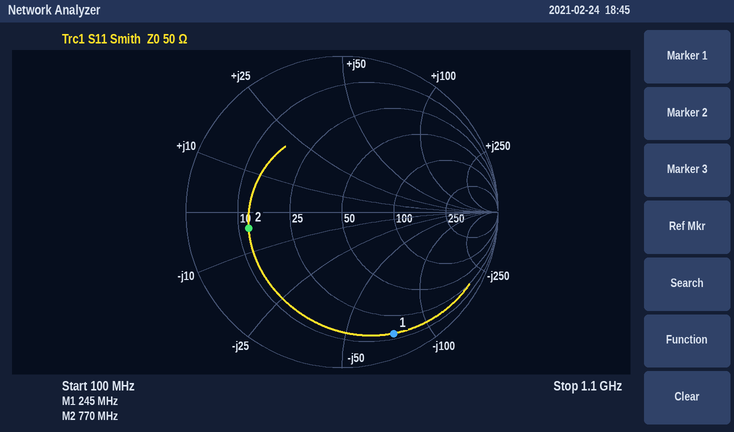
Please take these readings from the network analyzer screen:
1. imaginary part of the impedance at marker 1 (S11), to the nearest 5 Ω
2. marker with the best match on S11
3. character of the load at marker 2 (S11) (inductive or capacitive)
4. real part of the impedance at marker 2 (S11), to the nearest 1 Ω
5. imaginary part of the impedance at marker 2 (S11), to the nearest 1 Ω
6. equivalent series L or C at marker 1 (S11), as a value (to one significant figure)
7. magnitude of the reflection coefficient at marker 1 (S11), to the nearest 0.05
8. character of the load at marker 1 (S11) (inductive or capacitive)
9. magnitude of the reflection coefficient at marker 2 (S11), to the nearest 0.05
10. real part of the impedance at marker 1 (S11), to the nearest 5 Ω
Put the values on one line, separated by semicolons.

-75 Ω; marker 2; capacitive; 12 Ω; -4 Ω; 9 pF; 0.85; capacitive; 0.60; 15 Ω
